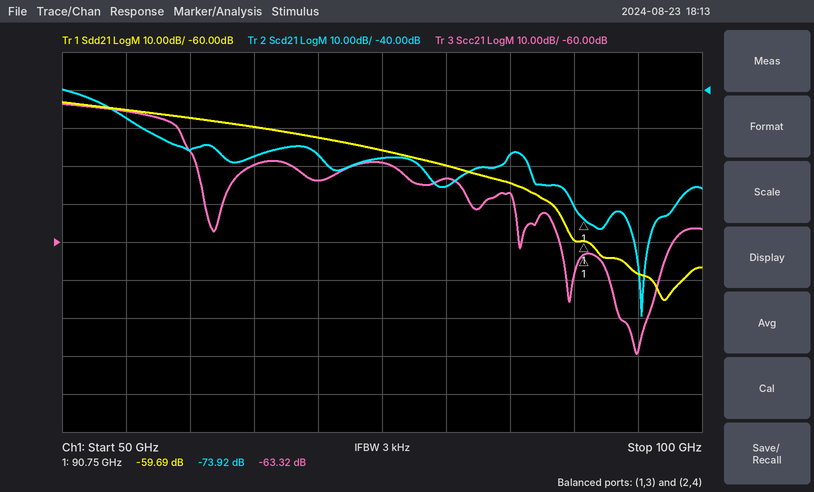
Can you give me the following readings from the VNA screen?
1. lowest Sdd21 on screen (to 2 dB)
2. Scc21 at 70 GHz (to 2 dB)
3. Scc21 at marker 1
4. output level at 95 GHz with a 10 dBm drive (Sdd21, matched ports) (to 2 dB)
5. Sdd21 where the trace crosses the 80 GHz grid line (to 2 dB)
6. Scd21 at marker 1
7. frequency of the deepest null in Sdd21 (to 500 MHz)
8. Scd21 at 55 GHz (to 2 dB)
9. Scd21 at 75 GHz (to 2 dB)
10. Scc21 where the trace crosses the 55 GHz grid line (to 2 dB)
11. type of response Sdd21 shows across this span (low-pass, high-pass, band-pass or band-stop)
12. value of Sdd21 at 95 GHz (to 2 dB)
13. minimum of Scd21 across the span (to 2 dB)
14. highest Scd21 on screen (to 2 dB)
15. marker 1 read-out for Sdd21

-76 dB
-44 dB
-63.32 dB
-58 dBm
-40 dB
-73.92 dB
97.0 GHz
-48 dB
-58 dB
-26 dB
low-pass
-68 dB
-100 dB
-40 dB
-59.69 dB
